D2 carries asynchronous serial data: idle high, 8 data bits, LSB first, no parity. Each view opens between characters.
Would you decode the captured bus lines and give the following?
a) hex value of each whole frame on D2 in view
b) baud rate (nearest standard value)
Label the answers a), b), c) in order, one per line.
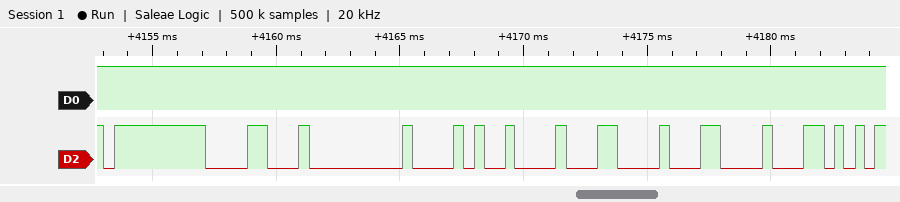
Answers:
a) FF, 18, 00, 28, 88, 88, 88
b) 2400 baud
